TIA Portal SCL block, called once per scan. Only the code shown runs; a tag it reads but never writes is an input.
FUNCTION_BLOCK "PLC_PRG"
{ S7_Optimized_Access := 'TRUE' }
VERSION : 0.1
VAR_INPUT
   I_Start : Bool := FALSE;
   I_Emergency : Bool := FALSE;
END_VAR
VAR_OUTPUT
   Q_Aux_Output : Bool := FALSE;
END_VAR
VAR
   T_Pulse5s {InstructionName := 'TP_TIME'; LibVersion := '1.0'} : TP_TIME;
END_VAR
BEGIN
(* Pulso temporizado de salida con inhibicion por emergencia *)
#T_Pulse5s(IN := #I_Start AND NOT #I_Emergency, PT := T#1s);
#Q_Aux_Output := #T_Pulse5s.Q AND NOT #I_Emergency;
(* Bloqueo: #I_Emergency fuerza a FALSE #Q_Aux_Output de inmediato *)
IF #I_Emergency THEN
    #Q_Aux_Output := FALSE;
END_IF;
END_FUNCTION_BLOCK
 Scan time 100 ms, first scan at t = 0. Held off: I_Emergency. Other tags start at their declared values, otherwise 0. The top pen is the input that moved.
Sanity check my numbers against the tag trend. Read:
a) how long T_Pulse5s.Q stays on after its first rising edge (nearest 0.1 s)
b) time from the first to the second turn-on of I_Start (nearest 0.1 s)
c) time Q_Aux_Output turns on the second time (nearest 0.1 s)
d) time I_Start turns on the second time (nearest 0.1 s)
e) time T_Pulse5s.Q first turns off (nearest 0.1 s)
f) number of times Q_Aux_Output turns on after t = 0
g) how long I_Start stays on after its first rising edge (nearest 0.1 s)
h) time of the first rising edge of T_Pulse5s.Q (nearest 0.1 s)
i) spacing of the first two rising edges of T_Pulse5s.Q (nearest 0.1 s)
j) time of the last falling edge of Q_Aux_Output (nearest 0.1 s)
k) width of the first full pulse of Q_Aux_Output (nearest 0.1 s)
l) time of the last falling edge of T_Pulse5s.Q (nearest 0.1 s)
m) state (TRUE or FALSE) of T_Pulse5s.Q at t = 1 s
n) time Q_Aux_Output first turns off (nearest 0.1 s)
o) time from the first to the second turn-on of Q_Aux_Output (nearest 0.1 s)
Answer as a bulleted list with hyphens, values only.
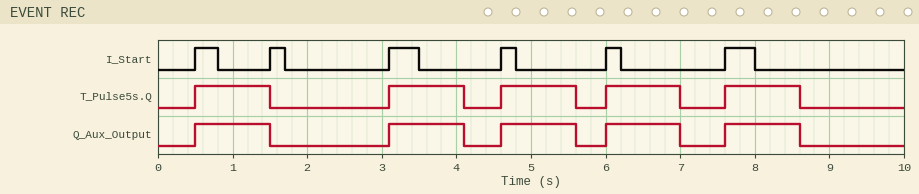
- 1.0 s
- 1.0 s
- 3.1 s
- 1.5 s
- 1.5 s
- 5
- 0.3 s
- 0.5 s
- 2.6 s
- 8.6 s
- 1.0 s
- 8.6 s
- TRUE
- 1.5 s
- 2.6 s
